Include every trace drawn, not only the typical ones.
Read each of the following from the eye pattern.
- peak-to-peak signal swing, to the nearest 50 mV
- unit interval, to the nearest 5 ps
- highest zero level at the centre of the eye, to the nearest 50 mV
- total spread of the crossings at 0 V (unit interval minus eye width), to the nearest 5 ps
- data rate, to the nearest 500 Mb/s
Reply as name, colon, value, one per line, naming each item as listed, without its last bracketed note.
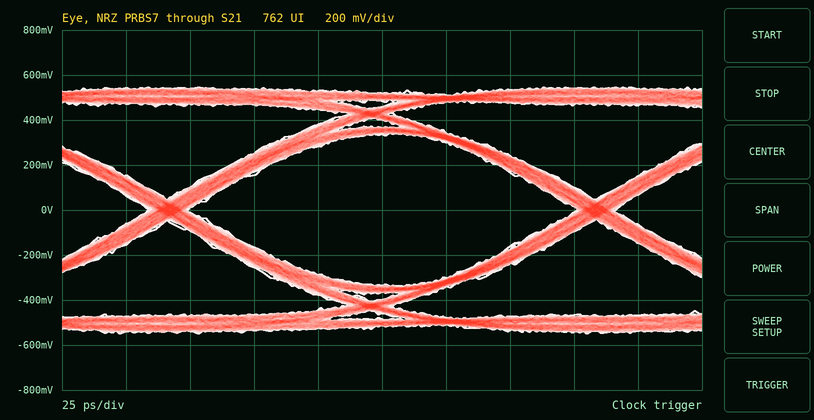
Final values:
peak-to-peak signal swing, to the nearest 50 mV: 1.10 V
unit interval, to the nearest 5 ps: 165 ps
highest zero level at the centre of the eye, to the nearest 50 mV: -350 mV
total spread of the crossings at 0 V (unit interval minus eye width), to the nearest 5 ps: 15 ps
data rate, to the nearest 500 Mb/s: 6.0 Gb/s
